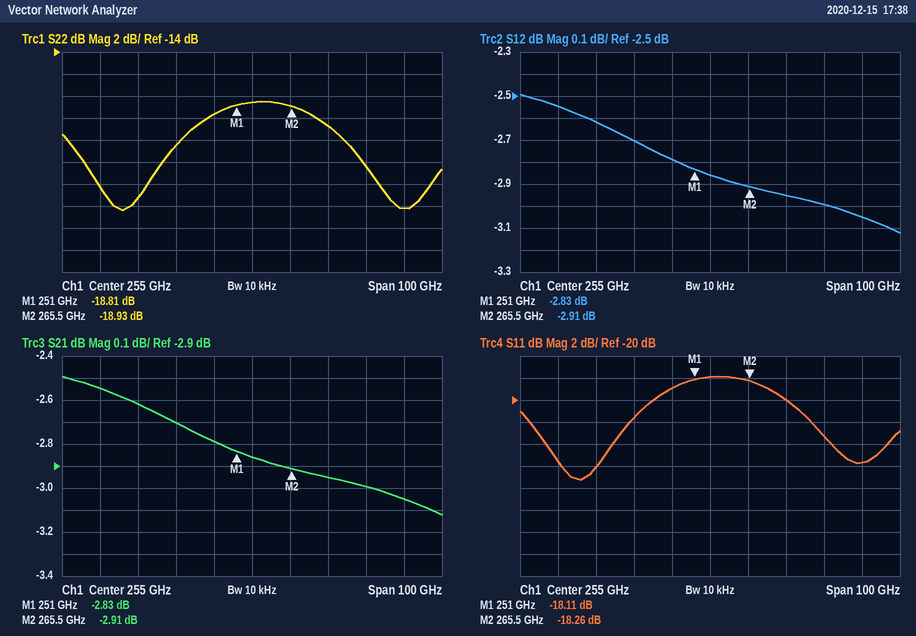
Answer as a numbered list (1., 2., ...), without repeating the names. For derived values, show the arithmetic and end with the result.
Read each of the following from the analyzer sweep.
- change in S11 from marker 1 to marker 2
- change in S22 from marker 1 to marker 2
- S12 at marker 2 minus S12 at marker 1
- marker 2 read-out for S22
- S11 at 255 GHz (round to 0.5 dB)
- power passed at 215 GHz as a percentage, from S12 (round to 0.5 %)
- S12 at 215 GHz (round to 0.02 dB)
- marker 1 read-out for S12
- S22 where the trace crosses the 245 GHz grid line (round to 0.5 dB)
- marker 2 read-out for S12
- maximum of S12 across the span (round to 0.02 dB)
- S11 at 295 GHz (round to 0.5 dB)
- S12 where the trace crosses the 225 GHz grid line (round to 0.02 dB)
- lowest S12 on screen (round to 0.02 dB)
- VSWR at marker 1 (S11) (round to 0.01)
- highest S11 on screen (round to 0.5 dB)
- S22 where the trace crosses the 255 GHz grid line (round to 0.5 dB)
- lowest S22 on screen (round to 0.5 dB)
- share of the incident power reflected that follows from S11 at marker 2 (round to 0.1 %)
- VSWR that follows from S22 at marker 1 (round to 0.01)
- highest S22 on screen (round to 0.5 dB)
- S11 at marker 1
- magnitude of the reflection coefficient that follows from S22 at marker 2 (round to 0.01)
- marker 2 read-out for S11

1. -18.26 − (-18.11) = -0.15 dB
2. -18.93 − (-18.81) = -0.12 dB
3. -2.91 − (-2.83) = -0.08 dB
4. -18.93 dB
5. -18.0 dB
6. 10^(-2.54/10) ≈ 55.7 %, so 55.5 % to the nearest 0.5 %
7. -2.54 dB
8. -2.83 dB
9. -19.5 dB
10. -2.91 dB
11. -2.50 dB
12. -25.5 dB
13. -2.62 dB
14. -3.12 dB
15. (1 + 0.1243)/(1 − 0.1243) ≈ 1.28
16. -18.0 dB
17. -18.5 dB
18. -28.5 dB
19. 10^(-18.26/10) ≈ 1.5 %
20. (1 + 0.1147)/(1 − 0.1147) ≈ 1.26
21. -18.5 dB
22. -18.11 dB
23. 10^(-18.93/20) ≈ 0.11
24. -18.26 dB
